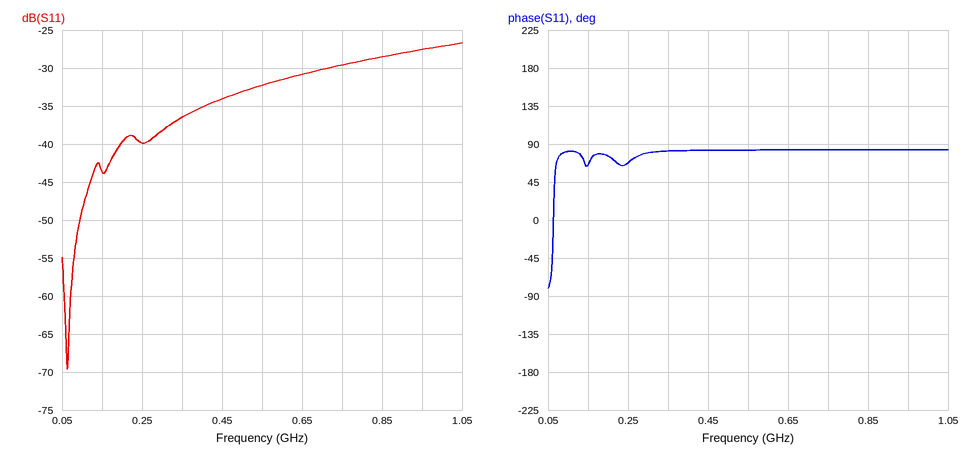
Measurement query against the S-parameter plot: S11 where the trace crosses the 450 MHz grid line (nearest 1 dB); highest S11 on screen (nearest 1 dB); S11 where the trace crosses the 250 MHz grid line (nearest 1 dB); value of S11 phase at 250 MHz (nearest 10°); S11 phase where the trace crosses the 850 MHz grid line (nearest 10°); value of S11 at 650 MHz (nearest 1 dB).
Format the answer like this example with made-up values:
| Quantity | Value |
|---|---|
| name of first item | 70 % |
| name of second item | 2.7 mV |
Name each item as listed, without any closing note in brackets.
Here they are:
| Quantity | Value |
|---|---|
| S11 where the trace crosses the 450 MHz grid line | -34 dB |
| highest S11 on screen | -27 dB |
| S11 where the trace crosses the 250 MHz grid line | -40 dB |
| value of S11 phase at 250 MHz | 70° |
| S11 phase where the trace crosses the 850 MHz grid line | 80° |
| value of S11 at 650 MHz | -31 dB |
